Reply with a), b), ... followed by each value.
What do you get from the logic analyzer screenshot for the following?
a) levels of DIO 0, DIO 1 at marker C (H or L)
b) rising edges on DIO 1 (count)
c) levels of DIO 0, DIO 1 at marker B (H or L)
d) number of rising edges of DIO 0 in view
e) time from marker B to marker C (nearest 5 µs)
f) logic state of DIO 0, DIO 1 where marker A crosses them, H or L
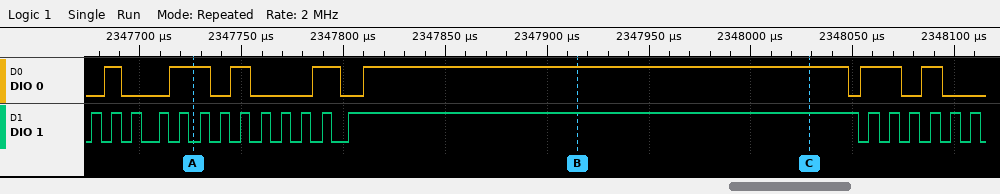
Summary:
a) DIO 0=H, DIO 1=H
b) 19
c) DIO 0=H, DIO 1=H
d) 7
e) 115 µs
f) DIO 0=H, DIO 1=L
